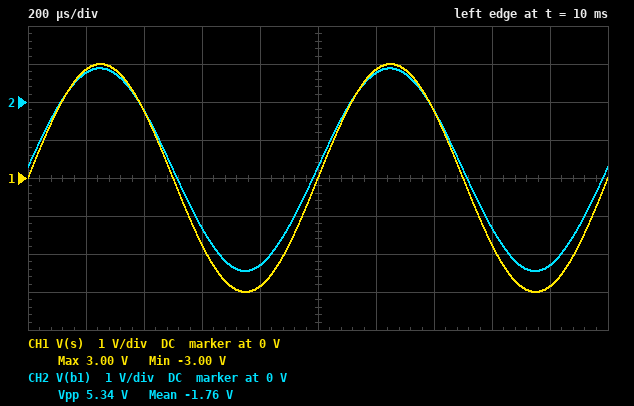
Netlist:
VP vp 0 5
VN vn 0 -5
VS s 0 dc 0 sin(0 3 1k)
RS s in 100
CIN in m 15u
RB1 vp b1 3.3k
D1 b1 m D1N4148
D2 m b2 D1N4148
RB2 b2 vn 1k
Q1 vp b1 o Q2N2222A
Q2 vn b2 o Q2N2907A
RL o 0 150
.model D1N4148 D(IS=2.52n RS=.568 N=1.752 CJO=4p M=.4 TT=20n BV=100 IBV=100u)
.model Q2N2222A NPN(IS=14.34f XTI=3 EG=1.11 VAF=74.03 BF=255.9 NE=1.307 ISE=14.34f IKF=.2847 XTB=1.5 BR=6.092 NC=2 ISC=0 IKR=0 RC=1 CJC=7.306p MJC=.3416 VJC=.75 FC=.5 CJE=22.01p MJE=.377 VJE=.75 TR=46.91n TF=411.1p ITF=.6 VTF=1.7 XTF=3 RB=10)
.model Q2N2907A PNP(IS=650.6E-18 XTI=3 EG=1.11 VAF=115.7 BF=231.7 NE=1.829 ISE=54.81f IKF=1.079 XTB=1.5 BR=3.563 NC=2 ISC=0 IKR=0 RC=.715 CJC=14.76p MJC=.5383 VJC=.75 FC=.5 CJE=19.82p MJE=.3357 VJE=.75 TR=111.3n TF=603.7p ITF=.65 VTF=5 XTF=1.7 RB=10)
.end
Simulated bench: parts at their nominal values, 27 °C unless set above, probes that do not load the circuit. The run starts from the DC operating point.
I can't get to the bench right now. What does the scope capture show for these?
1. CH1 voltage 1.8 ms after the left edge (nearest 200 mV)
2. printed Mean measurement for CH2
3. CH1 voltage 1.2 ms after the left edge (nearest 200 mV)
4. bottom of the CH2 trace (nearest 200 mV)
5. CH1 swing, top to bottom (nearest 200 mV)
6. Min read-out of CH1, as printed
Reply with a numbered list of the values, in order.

1. -2.8 V
2. -1.76 V
3. 2.8 V
4. -4.4 V
5. 6.0 V
6. -3.00 V
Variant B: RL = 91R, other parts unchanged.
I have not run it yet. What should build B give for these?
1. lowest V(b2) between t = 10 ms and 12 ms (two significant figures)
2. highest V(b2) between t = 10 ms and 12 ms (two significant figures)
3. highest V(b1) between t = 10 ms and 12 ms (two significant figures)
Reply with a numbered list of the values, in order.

1. -4.8 V
2. -340 mV
3. 910 mV
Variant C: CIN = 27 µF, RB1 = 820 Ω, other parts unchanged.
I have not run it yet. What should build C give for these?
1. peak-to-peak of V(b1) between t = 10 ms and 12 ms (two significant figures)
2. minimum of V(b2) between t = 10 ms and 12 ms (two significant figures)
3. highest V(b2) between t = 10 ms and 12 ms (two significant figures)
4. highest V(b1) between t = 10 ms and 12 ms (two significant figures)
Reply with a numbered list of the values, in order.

1. 4.8 V
2. -2.7 V
3. 2.2 V
4. 3.5 V
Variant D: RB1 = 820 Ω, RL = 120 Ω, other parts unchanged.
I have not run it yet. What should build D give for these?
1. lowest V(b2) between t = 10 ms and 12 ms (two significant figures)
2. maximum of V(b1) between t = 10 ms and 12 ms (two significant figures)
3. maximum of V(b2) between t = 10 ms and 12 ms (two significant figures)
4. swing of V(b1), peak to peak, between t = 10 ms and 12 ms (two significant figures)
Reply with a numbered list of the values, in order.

1. -2.7 V
2. 3.5 V
3. 2.2 V
4. 4.8 V
